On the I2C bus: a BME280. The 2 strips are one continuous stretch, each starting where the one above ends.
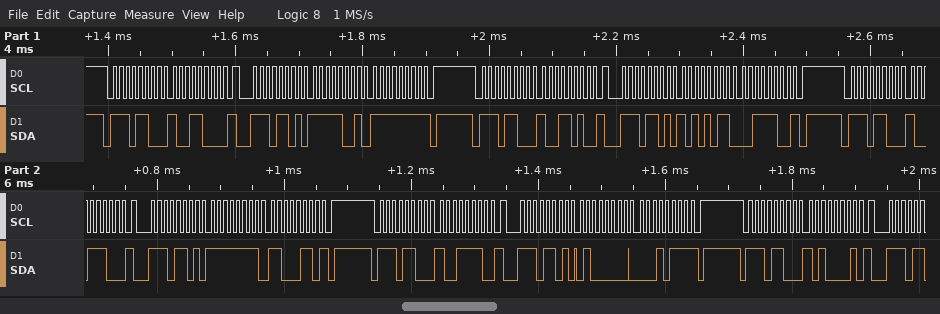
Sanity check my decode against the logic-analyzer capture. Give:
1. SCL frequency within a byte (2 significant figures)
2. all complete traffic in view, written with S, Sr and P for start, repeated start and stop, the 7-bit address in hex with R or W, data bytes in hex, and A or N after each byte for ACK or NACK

100 kHz
S 76W A 98 A Sr 76R A F9 A FF N P S 76W A 9A A Sr 76R A AB A 3C N P S 76W A 9C A Sr 76R A FF A C6 N P S 76W A 9E A Sr 76R A 40 A 17 N P S 76W A A1 A
